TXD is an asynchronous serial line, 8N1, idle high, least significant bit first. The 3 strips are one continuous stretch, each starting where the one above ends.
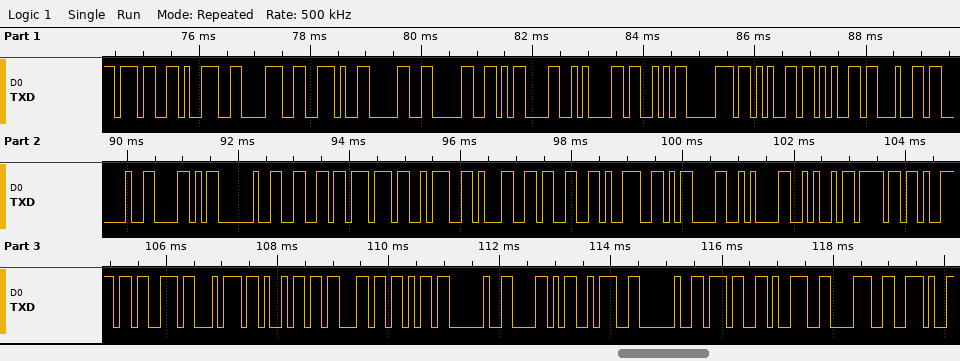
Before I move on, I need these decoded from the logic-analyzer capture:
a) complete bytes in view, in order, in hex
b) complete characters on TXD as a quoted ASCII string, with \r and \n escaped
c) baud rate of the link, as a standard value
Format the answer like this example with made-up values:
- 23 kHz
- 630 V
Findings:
- 37 39 38 2E 30 30 0D 0A 53 70 65 65 64 20 58 20 66 77 3A 31 33 39 0D 0A 4A 6F 79 73 74 69 63 6B 20 58 3A 20 37 39 38 2E
- "798.00\r\nSpeed X fw:139\r\nJoystick X: 798."
- 9600 baud
